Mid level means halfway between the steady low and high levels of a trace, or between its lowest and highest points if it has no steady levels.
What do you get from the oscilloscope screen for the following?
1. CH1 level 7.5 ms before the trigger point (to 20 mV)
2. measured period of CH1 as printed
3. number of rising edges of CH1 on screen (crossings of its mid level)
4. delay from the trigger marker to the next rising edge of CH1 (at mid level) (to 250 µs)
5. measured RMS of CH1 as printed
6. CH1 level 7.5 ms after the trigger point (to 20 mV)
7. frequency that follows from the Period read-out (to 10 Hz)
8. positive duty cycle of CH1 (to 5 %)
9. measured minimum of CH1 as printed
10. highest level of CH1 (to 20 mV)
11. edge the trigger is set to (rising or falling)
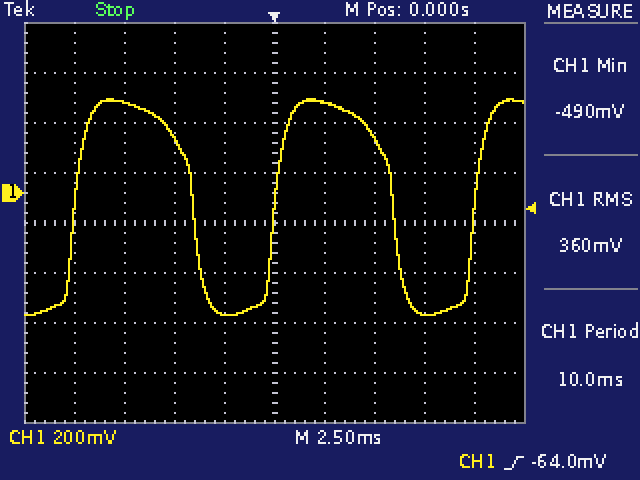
360 mV
10.0 ms
3
10.00 ms
360 mV
-480 mV
100 Hz
60 %
-490 mV
380 mV
rising
